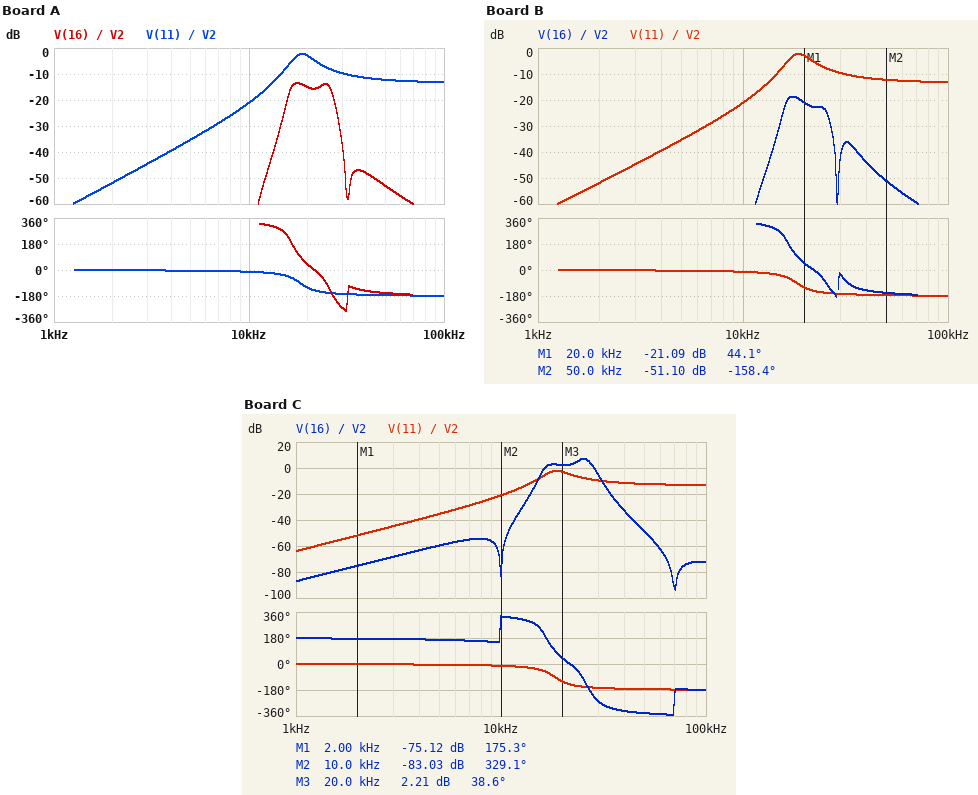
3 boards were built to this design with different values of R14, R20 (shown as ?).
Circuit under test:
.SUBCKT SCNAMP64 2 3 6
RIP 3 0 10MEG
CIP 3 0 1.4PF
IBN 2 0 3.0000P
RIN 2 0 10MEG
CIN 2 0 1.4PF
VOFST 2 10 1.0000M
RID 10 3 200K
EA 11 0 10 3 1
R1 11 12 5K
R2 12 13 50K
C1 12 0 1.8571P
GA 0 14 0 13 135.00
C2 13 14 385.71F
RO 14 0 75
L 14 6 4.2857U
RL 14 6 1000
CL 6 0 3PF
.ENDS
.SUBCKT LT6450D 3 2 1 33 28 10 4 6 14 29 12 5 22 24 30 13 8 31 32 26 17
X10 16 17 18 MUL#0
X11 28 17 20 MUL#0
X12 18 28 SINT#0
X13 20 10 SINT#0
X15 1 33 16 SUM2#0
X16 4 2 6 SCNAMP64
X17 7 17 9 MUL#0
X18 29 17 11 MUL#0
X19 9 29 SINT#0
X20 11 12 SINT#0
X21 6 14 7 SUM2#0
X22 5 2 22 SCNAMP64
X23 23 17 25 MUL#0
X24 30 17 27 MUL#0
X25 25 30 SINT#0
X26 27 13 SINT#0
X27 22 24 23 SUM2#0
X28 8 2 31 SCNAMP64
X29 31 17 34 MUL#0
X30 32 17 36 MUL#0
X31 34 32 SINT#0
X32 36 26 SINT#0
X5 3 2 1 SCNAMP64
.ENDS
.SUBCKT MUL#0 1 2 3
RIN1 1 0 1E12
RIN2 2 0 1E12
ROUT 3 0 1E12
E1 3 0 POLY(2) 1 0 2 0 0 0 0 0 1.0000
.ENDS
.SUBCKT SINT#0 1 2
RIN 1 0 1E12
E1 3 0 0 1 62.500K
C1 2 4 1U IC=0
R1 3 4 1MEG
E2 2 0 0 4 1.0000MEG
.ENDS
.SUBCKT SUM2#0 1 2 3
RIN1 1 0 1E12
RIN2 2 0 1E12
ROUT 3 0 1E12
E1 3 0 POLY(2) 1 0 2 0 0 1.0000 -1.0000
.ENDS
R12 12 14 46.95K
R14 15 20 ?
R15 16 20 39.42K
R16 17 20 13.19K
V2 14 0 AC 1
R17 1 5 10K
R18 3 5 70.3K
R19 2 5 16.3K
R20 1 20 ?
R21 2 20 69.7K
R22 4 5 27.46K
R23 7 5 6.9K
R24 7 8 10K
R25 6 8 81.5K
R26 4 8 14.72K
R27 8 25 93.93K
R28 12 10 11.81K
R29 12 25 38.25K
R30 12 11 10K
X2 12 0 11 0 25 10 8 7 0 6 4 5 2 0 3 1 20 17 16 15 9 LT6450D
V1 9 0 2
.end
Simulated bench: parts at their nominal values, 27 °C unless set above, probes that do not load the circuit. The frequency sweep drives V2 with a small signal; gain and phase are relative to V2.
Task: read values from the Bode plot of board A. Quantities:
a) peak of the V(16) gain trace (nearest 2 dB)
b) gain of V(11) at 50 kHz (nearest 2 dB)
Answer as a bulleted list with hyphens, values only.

- -14 dB
- -12 dB
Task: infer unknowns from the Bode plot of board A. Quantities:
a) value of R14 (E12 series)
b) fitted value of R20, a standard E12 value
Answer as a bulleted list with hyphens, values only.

- 6.8 kΩ
- 27 kΩ
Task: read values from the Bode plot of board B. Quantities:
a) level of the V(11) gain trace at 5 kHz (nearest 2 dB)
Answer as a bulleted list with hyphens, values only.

- -36 dB
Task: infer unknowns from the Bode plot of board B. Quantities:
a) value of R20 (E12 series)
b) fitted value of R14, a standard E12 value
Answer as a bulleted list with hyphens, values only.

- 33 kΩ
- 5.6 kΩ
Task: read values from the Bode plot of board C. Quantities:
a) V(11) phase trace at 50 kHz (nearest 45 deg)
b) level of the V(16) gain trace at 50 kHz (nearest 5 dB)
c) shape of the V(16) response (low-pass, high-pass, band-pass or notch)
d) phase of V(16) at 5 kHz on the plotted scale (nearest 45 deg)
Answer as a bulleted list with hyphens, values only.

- -180 deg
- -50 dB
- band-pass
- 180 deg
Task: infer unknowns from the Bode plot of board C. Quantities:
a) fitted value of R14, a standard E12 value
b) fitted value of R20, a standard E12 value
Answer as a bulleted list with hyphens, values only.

- 6.8 kΩ
- 5.6 kΩ
